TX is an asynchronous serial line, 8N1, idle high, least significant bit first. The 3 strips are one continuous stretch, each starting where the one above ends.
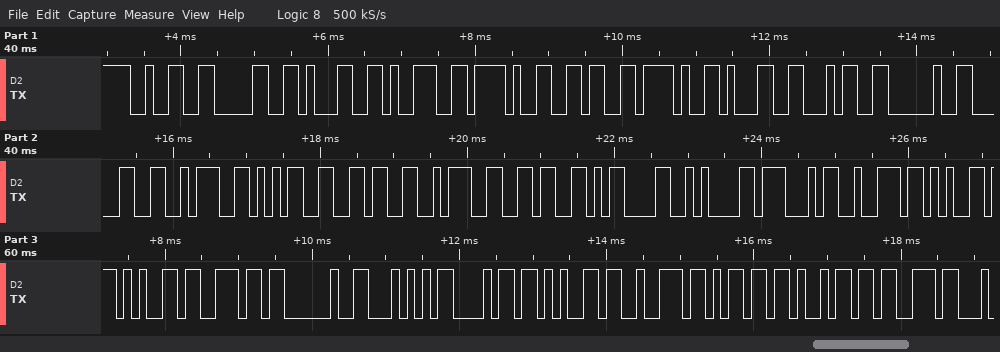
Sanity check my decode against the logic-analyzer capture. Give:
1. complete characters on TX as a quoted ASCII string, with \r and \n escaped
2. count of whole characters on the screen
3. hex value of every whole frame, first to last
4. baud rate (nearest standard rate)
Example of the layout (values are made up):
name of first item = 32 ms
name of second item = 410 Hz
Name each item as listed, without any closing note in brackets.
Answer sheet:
complete characters on TX as a quoted ASCII string, with \r and \n escaped = "2019/6/14 0:56:6\r\nGreen Thermis"
count of whole characters on the screen = 31
hex value of every whole frame, first to last = 32 30 31 39 2F 36 2F 31 34 20 30 3A 35 36 3A 36 0D 0A 47 72 65 65 6E 20 54 68 65 72 6D 69 73
baud rate = 9600 baud
